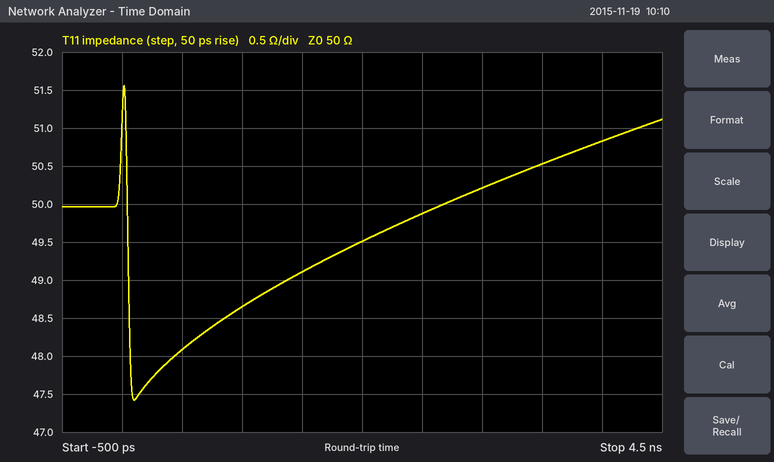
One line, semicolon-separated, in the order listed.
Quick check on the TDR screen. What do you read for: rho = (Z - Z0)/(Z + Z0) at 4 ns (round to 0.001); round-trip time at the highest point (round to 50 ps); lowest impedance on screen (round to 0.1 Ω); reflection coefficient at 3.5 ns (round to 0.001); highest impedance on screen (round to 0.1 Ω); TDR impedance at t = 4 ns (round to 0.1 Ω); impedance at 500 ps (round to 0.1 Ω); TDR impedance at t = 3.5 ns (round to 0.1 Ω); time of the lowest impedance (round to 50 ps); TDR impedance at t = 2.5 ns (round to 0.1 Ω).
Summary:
+0.008; 0 ps; 47.4 Ω; +0.005; 51.6 Ω; 50.8 Ω; 48.1 Ω; 50.5 Ω; 100 ps; 49.9 Ω
